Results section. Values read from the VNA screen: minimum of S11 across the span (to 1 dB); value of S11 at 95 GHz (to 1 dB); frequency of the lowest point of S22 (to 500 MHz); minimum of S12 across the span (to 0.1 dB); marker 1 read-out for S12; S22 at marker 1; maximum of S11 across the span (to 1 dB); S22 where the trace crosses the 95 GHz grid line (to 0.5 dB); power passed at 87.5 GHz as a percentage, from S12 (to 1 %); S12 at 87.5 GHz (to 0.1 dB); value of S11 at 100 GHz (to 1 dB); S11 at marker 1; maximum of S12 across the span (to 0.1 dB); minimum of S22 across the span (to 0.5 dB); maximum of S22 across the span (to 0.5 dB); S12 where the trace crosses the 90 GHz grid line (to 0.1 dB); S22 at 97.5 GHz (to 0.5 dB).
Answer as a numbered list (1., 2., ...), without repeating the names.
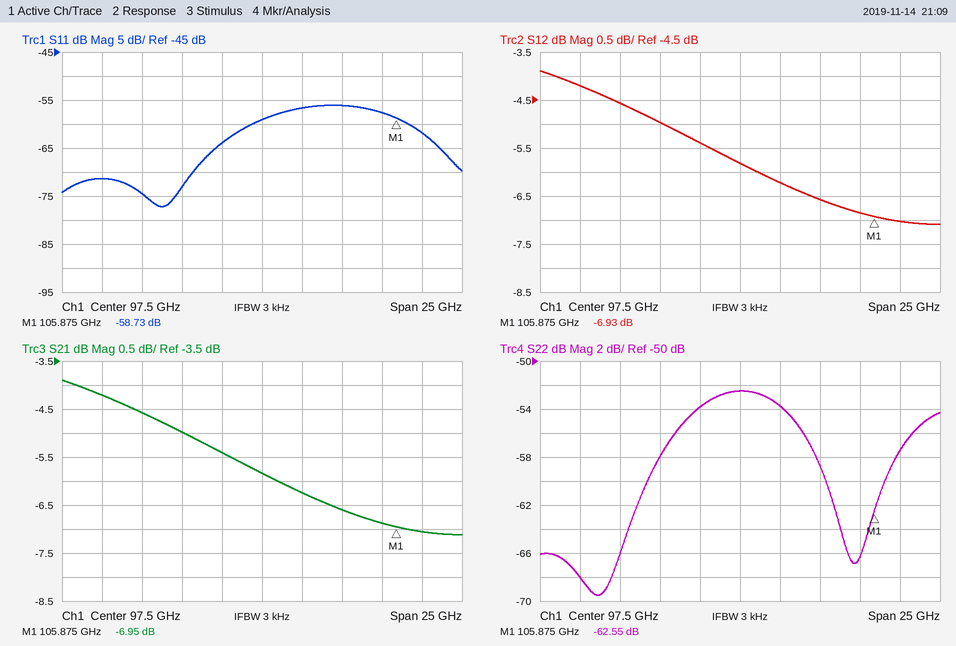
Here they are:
1. -77 dB
2. -64 dB
3. 88.5 GHz
4. -7.1 dB
5. -6.93 dB
6. -62.55 dB
7. -56 dB
8. -54.0 dB
9. 38 %
10. -4.2 dB
11. -57 dB
12. -58.73 dB
13. -3.9 dB
14. -69.5 dB
15. -52.5 dB
16. -4.6 dB
17. -52.5 dB
